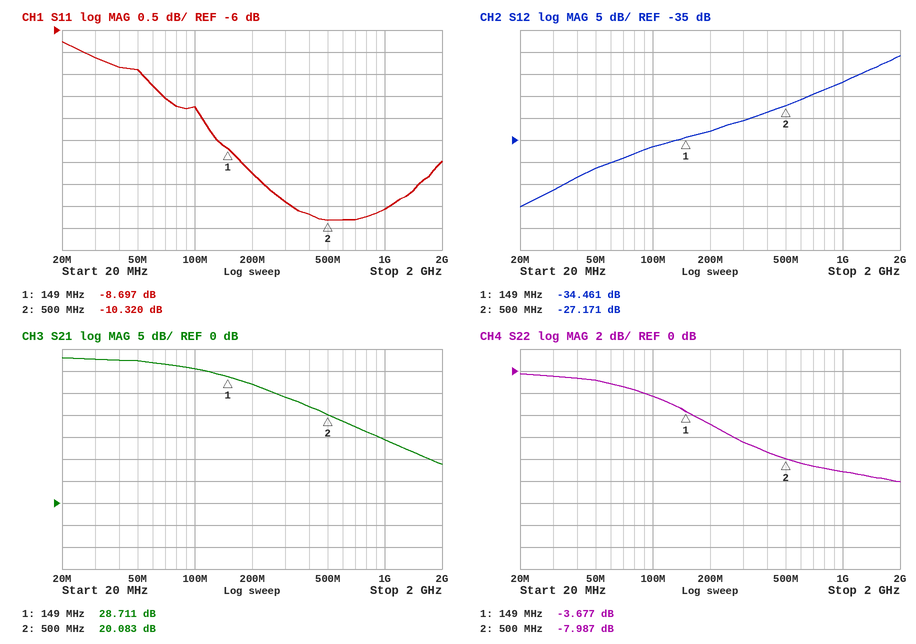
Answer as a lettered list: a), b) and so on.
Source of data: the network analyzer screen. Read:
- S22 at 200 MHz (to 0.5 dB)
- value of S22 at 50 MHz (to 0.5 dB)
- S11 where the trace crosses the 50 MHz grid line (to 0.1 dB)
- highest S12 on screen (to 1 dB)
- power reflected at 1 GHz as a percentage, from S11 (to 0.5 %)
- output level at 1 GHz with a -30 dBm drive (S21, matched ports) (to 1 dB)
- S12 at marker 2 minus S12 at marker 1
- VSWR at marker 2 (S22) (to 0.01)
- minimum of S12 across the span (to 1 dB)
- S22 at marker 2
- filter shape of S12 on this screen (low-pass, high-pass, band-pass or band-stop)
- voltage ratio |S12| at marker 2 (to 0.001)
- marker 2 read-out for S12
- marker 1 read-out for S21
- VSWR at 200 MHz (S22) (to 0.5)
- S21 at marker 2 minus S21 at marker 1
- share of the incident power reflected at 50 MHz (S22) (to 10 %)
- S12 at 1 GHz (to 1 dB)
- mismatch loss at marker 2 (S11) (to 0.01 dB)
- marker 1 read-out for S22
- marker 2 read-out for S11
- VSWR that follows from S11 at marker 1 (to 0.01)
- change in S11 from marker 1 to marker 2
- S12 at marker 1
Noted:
a) -5.0 dB
b) -1.0 dB
c) -6.9 dB
d) -16 dB
e) 10.0 %
f) -16 dBm
g) 7.290 dB
h) 2.33
i) -50 dB
j) -7.987 dB
k) high-pass
l) 0.044
m) -27.171 dB
n) 28.711 dB
o) 3.5
p) -8.628 dB
q) 80 %
r) -22 dB
s) 0.42 dB
t) -3.677 dB
u) -10.320 dB
v) 2.16
w) -1.623 dB
x) -34.461 dB
